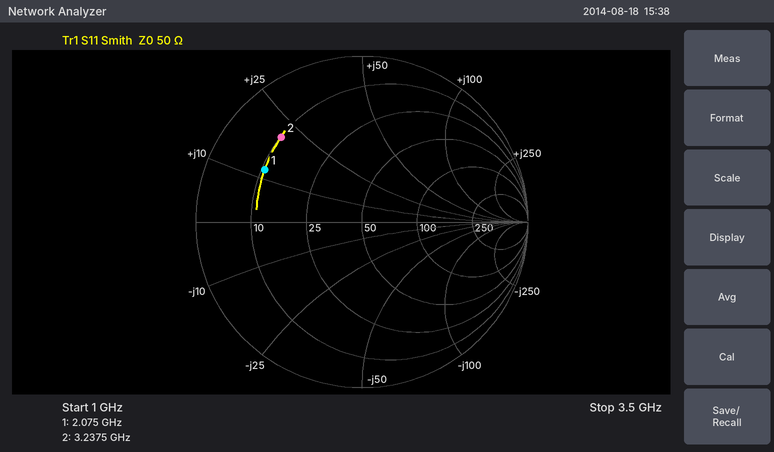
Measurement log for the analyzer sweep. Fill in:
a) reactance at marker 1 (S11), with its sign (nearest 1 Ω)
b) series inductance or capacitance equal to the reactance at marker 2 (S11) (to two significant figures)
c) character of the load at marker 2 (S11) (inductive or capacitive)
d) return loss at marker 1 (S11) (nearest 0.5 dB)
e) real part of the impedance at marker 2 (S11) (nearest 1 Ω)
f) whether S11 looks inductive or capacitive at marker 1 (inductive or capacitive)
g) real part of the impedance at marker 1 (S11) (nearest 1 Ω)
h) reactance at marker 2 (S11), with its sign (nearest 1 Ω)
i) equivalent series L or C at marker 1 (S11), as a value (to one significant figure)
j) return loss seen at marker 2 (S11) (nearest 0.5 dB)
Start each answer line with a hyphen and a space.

- +12 Ω
- 1.0 nH
- inductive
- 3.5 dB
- 10 Ω
- inductive
- 11 Ω
- +21 Ω
- 900 pH
- 3.0 dB
